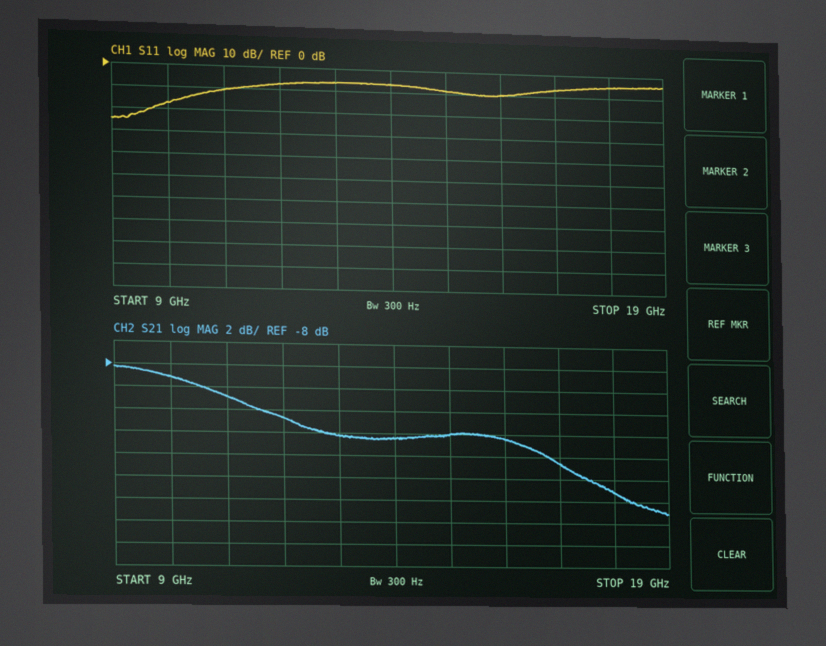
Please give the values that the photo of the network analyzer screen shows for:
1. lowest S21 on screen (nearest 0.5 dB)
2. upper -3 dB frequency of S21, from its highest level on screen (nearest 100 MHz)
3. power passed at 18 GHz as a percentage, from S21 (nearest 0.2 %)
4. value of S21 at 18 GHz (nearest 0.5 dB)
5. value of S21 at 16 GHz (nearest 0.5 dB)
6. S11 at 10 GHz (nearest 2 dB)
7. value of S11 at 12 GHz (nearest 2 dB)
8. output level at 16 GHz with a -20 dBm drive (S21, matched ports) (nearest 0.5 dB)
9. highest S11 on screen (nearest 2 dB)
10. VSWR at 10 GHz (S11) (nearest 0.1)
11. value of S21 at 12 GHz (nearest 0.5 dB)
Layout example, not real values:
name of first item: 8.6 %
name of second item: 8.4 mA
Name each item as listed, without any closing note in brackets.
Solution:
lowest S21 on screen: -21.0 dB
upper -3 dB frequency of S21, from its highest level on screen: 11.2 GHz
power passed at 18 GHz as a percentage, from S21: 1.2 %
value of S21 at 18 GHz: -19.0 dB
value of S21 at 16 GHz: -14.5 dB
S11 at 10 GHz: -18 dB
value of S11 at 12 GHz: -8 dB
output level at 16 GHz with a -20 dBm drive (S21, matched ports): -34.5 dBm
highest S11 on screen: -4 dB
VSWR at 10 GHz (S11): 1.3
value of S21 at 12 GHz: -12.5 dB
